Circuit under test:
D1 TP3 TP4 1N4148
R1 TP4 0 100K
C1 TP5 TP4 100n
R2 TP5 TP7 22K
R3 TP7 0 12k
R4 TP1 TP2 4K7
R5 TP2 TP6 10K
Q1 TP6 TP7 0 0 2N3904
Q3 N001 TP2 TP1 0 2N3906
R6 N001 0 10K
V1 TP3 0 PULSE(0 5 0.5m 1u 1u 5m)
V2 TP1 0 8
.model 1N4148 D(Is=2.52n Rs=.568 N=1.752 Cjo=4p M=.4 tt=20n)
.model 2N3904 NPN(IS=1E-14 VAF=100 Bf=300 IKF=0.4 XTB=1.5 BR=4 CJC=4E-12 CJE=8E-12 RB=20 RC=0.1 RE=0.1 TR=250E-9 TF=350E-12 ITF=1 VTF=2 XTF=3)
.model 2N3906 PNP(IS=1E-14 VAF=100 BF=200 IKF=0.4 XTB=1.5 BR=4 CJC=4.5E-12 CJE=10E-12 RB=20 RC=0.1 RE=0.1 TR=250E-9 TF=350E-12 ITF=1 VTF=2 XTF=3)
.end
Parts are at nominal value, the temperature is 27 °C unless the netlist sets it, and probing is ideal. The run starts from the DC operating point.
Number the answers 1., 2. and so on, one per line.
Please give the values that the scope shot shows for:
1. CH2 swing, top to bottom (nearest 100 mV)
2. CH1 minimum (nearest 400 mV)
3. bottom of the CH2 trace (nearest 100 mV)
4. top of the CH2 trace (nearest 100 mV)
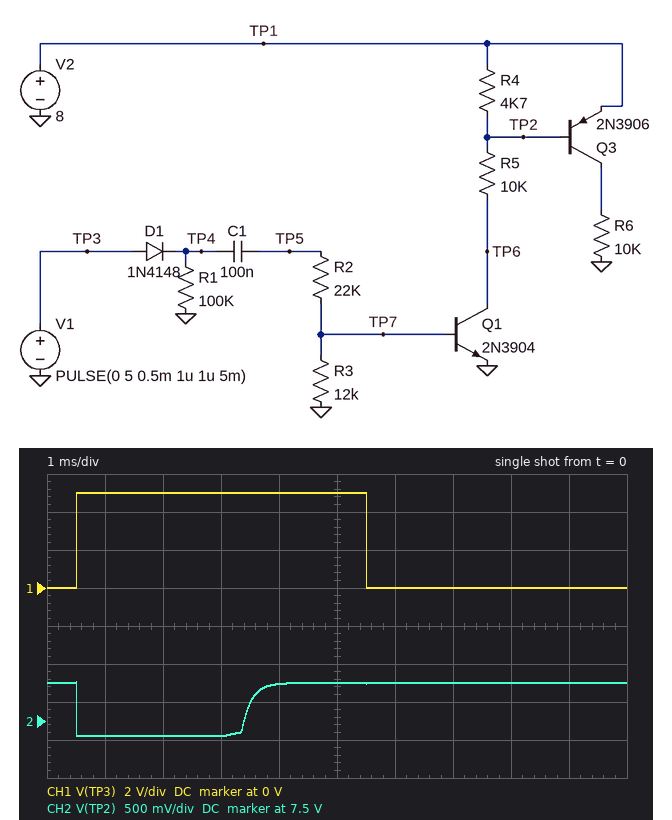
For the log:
1. 700 mV
2. 0 V
3. 7.3 V
4. 8.0 V
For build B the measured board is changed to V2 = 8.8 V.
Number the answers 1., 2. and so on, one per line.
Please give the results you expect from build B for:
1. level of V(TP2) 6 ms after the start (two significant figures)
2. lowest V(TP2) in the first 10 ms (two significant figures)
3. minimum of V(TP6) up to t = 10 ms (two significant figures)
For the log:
1. 8.8 V
2. 8.1 V
3. 29 mV
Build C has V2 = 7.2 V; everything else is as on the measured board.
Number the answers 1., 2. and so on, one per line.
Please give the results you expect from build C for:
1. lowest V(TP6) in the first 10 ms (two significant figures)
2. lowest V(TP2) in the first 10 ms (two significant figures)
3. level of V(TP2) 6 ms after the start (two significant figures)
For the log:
1. 26 mV
2. 6.5 V
3. 7.2 V
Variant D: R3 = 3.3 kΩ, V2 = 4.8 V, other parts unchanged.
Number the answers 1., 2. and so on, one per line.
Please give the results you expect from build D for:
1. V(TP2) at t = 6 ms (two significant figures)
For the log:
1. 4.8 V
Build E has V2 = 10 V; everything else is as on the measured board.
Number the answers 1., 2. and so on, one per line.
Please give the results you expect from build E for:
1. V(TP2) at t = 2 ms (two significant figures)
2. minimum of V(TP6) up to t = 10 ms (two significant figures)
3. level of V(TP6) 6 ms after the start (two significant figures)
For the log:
1. 9.3 V
2. 31 mV
3. 10 V
